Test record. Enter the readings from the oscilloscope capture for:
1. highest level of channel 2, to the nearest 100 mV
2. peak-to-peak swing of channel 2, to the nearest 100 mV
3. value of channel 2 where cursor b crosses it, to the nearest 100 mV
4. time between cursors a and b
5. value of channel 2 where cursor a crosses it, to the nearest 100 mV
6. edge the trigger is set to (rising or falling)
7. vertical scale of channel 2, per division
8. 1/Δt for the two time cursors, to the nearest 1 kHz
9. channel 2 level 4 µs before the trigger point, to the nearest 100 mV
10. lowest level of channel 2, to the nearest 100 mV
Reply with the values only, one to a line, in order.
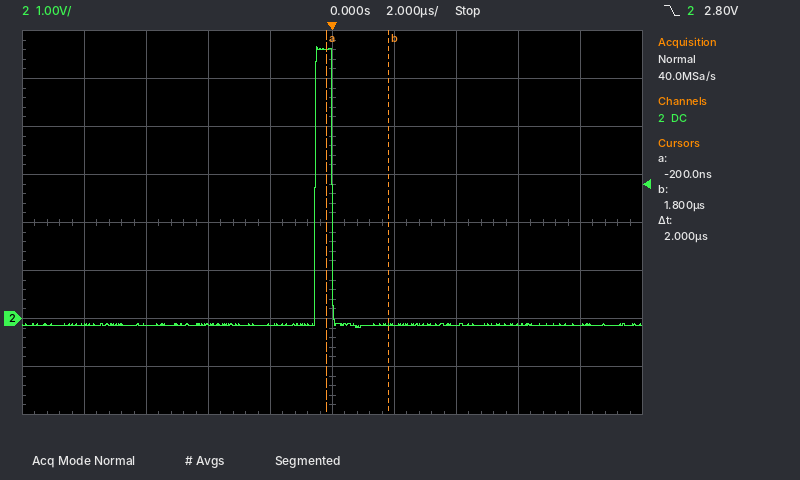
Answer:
5.7 V
5.9 V
-100 mV
2 µs
5.6 V
falling
1 V
500 kHz
-100 mV
-200 mV
